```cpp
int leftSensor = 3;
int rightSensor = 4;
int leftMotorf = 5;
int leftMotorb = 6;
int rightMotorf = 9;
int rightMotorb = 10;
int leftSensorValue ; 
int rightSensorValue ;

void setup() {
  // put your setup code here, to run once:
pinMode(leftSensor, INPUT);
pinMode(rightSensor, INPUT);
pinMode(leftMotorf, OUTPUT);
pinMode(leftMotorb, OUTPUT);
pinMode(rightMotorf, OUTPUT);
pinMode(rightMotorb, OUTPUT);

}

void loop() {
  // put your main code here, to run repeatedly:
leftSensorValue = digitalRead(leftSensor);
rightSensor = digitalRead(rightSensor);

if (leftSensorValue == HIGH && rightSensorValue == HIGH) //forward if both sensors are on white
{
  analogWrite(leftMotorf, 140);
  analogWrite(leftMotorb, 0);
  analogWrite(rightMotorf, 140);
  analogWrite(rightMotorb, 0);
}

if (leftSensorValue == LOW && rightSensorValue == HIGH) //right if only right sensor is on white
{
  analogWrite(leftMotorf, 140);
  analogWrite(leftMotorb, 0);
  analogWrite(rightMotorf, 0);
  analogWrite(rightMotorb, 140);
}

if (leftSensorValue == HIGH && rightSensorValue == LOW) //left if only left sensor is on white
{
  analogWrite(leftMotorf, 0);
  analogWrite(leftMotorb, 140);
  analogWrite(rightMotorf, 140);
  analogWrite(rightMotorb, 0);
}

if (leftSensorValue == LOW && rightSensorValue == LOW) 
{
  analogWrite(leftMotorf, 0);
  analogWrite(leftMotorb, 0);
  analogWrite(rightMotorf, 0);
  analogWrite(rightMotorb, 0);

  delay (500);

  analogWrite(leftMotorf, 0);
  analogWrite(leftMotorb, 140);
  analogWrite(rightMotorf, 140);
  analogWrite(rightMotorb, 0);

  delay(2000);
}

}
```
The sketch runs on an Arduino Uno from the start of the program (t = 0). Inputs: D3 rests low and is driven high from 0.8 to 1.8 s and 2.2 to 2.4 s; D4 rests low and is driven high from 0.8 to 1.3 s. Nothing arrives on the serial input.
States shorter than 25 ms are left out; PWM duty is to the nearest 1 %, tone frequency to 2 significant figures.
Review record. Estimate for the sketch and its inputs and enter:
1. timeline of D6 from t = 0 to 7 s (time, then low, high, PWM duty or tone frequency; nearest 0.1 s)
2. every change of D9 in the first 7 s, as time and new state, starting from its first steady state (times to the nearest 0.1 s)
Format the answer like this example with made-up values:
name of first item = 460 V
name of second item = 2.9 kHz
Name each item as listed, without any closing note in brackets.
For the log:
timeline of D6 from t = 0 to 7 s = 0 s low; 0.5 s PWM 55 %; 2.5 s low; 3 s PWM 55 %; 5 s low; 5.5 s PWM 55 %
every change of D9 in the first 7 s, as time and new state, starting from its first steady state = 0 s low; 0.5 s PWM 55 %; 2.5 s low; 3 s PWM 55 %; 5 s low; 5.5 s PWM 55 %
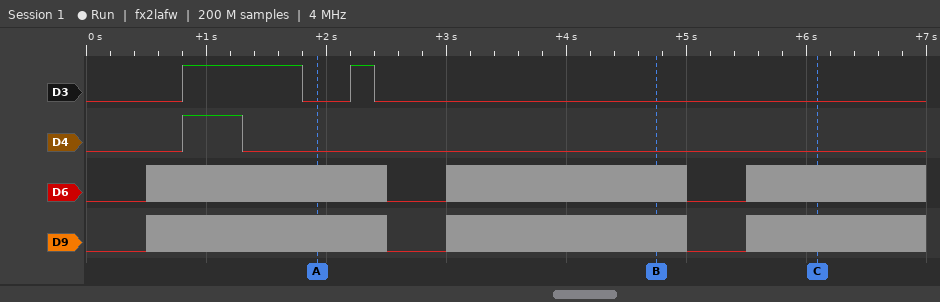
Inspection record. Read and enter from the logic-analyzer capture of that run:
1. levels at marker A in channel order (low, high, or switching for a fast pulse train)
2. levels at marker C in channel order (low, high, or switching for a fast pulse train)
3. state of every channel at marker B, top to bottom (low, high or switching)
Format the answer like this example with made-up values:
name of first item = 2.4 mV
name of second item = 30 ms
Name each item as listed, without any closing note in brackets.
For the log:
levels at marker A in channel order = D3 low, D4 low, D6 switching, D9 switching
levels at marker C in channel order = D3 low, D4 low, D6 switching, D9 switching
state of every channel at marker B, top to bottom = D3 low, D4 low, D6 switching, D9 switching
